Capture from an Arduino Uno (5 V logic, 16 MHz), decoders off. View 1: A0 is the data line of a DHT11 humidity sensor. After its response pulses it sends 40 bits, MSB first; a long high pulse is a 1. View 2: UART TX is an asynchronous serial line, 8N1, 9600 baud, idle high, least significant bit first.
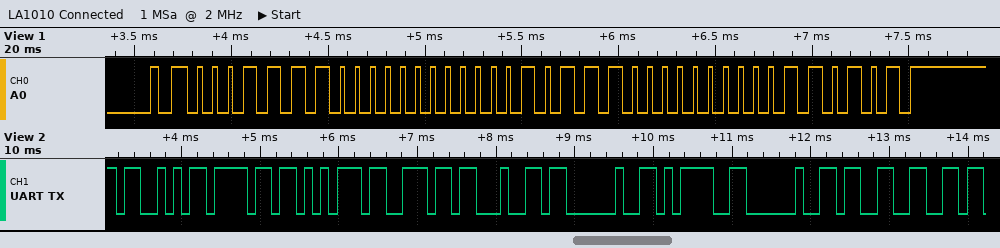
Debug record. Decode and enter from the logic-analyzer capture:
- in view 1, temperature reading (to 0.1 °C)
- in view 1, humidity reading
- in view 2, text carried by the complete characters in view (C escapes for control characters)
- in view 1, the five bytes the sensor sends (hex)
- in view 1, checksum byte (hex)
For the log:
23.0 °C
30 %
"Sound = 3"
1E 00 17 00 35
0x35
